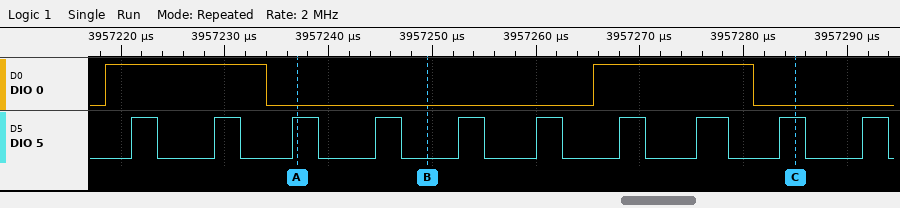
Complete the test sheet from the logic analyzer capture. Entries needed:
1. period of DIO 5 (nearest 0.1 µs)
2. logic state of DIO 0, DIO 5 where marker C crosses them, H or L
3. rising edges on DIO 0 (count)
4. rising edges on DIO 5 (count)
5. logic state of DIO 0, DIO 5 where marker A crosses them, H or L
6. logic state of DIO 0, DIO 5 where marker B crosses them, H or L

7.8 µs
DIO 0=L, DIO 5=H
2
10
DIO 0=L, DIO 5=H
DIO 0=L, DIO 5=L
